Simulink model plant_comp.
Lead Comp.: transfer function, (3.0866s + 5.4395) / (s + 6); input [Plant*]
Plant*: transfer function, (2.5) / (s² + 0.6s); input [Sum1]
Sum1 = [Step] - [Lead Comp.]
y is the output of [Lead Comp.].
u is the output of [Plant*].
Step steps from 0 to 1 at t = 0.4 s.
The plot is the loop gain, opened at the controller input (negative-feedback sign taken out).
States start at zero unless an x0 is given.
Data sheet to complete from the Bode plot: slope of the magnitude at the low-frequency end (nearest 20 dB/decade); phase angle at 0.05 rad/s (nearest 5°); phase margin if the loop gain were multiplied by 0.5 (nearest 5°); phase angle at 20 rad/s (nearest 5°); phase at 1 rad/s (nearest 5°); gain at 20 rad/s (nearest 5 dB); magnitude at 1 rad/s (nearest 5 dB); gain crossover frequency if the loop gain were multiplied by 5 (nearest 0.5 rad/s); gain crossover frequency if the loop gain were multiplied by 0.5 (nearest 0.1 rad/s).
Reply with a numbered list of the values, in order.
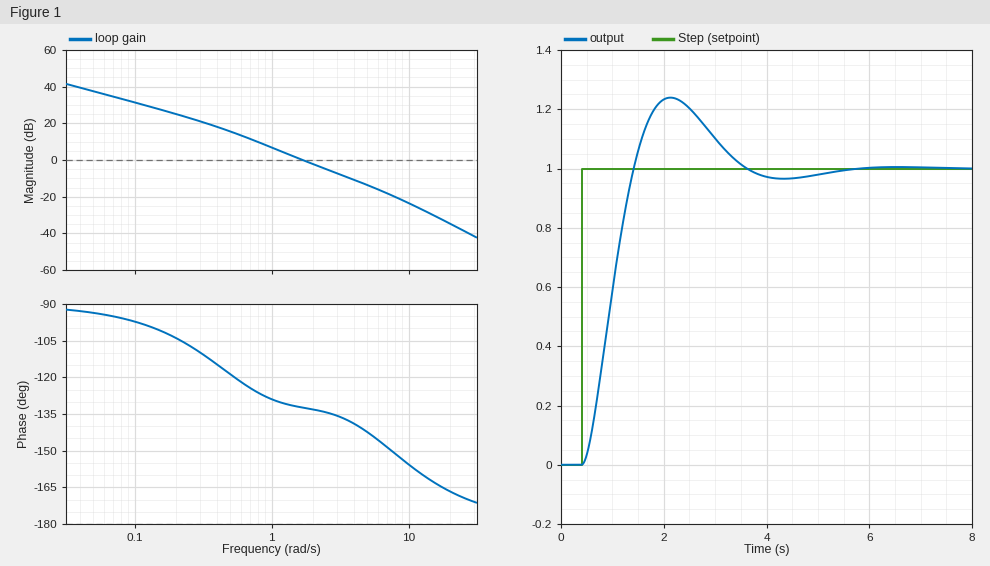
1. -20 dB/decade
2. -95°
3. 50°
4. -165°
5. -130°
6. -35 dB
7. 5 dB
8. 5.0 rad/s
9. 1.1 rad/s
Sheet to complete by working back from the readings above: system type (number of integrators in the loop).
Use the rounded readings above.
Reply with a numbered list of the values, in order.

1. 1
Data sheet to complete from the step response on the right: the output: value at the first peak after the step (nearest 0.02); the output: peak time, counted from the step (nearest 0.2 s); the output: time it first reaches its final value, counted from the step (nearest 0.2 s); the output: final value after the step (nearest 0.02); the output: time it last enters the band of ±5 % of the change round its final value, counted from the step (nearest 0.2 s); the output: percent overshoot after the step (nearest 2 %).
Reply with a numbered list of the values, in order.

1. 1.24
2. 1.8 s
3. 1.0 s
4. 1.00
5. 2.8 s
6. 24 %
